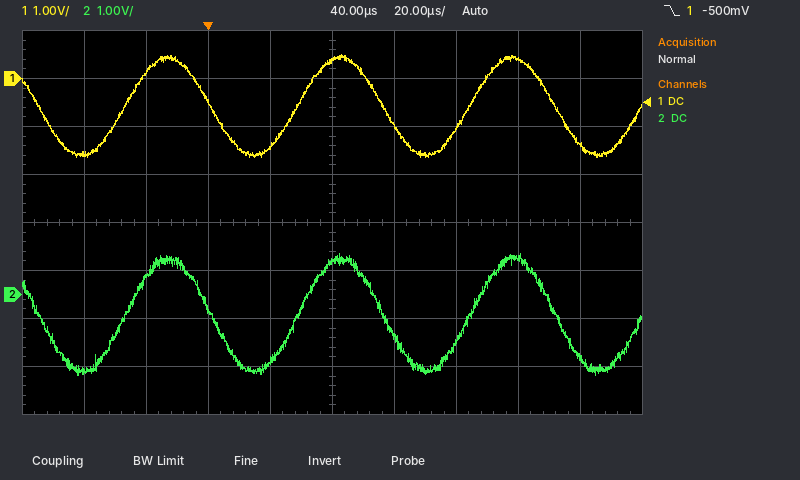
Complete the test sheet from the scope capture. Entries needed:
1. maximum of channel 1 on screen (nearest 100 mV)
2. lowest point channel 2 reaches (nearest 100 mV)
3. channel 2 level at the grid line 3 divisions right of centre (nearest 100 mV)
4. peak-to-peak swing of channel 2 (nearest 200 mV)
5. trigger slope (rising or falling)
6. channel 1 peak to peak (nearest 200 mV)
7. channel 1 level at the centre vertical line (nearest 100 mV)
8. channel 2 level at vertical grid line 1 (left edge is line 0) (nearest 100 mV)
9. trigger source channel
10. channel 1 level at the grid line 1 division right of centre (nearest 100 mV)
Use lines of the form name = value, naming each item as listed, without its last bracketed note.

maximum of channel 1 on screen = 500 mV
lowest point channel 2 reaches = -1.7 V
channel 2 level at the grid line 3 divisions right of centre = 800 mV
peak-to-peak swing of channel 2 = 2.6 V
trigger slope = falling
channel 1 peak to peak = 2.2 V
channel 1 level at the centre vertical line = 400 mV
channel 2 level at vertical grid line 1 (left edge is line 0) = -1.6 V
trigger source channel = channel 1
channel 1 level at the grid line 1 division right of centre = -1.0 V
